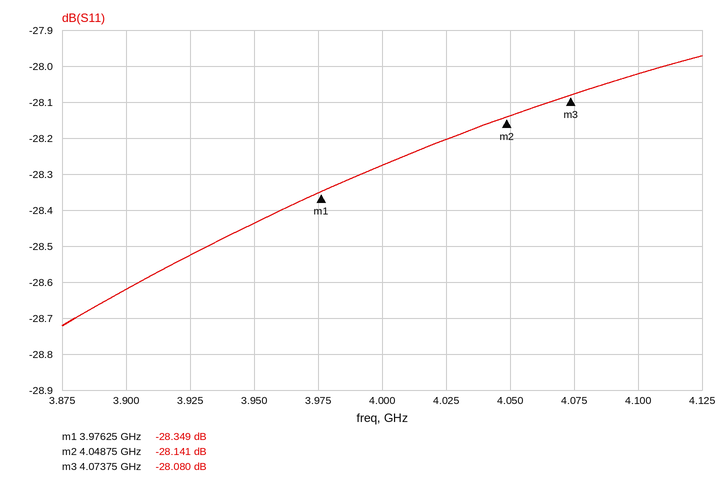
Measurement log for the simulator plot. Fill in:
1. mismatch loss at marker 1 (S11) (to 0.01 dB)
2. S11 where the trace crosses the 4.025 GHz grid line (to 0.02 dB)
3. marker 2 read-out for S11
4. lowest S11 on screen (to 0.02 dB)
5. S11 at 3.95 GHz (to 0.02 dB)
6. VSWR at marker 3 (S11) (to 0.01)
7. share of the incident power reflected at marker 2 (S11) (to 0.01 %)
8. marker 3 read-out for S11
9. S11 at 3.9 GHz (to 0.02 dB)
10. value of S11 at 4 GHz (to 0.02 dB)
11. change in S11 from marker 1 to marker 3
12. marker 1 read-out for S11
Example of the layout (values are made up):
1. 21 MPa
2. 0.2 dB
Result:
1. 0.01 dB
2. -28.20 dB
3. -28.141 dB
4. -28.72 dB
5. -28.44 dB
6. 1.08
7. 0.15 %
8. -28.080 dB
9. -28.62 dB
10. -28.28 dB
11. 0.269 dB
12. -28.349 dB
